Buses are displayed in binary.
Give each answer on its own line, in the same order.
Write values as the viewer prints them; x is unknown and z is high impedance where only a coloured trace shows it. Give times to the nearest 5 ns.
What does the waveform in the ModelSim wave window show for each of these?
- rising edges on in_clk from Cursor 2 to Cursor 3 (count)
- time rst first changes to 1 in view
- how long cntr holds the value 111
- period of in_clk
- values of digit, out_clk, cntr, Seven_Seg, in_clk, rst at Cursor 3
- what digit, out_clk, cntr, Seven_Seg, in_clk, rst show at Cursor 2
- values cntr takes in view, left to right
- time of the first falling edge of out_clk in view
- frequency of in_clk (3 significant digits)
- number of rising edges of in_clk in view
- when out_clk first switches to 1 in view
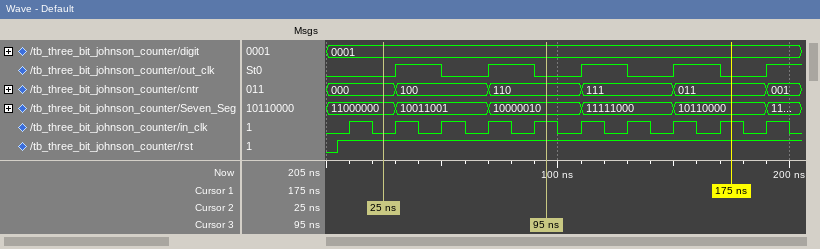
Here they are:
4
5 ns
40 ns
20 ns
digit=0001, out_clk=0, cntr=110, Seven_Seg=10000010, in_clk=1, rst=1
digit=0001, out_clk=0, cntr=000, Seven_Seg=11000000, in_clk=0, rst=1
000, 100, 110, 111, 011, 001
50 ns
50.0 MHz
10
30 ns
